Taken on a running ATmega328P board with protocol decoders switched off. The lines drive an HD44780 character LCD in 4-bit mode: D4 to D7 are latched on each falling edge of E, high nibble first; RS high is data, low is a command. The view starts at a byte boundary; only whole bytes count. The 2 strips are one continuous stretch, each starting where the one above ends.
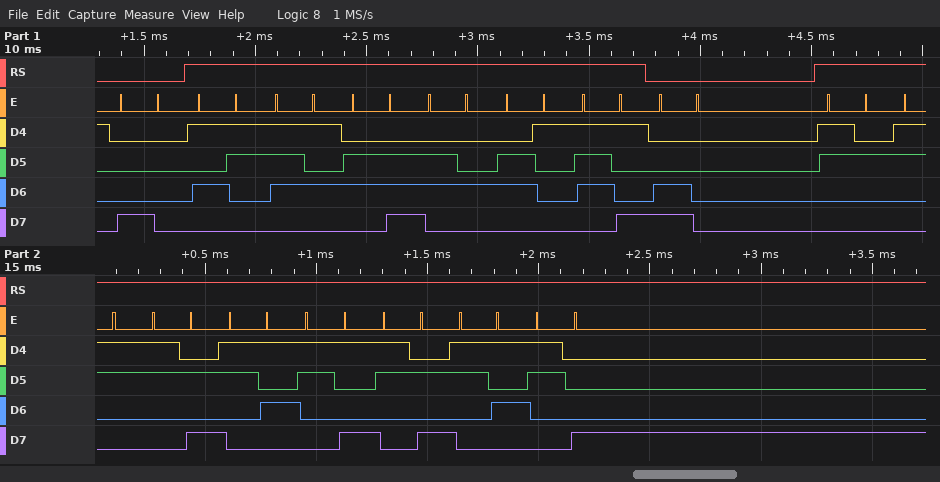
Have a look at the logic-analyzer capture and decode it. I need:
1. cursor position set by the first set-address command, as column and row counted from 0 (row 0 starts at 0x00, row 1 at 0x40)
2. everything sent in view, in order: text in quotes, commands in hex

column 0, row 0
0x80 "Sunday" 0xC0 "23:59:58"
